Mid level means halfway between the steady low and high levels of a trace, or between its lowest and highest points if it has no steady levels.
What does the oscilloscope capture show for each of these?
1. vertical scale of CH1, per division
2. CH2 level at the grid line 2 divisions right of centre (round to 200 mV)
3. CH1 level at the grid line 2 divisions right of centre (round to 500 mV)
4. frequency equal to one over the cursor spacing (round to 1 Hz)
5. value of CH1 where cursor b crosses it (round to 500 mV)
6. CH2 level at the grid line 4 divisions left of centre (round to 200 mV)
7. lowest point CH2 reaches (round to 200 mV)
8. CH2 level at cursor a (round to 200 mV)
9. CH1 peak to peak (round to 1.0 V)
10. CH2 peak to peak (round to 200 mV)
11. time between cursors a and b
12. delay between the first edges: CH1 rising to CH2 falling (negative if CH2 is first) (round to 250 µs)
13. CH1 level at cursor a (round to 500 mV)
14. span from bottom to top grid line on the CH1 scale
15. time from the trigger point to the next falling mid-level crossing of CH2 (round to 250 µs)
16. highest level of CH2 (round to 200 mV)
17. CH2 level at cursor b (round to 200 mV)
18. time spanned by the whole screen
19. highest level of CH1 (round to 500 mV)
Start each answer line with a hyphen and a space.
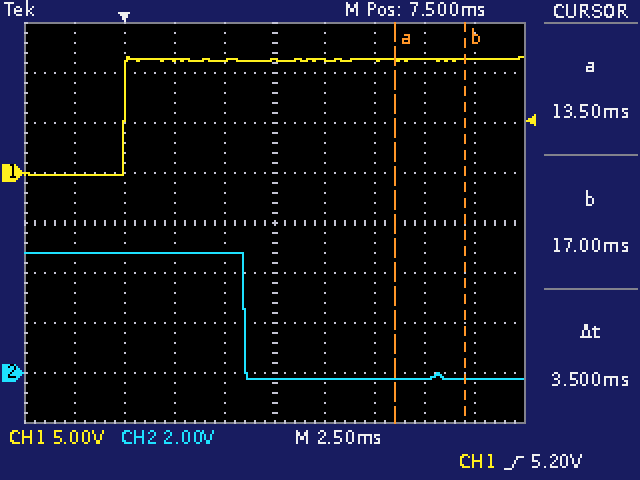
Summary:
- 5 V
- -200 mV
- 11.5 V
- 286 Hz
- 11.5 V
- 4.8 V
- -200 mV
- -200 mV
- 12.0 V
- 5.0 V
- 3.5 ms
- +6.00 ms
- 11.5 V
- 40 V
- 6.00 ms
- 4.8 V
- -200 mV
- 25 ms
- 11.5 V
